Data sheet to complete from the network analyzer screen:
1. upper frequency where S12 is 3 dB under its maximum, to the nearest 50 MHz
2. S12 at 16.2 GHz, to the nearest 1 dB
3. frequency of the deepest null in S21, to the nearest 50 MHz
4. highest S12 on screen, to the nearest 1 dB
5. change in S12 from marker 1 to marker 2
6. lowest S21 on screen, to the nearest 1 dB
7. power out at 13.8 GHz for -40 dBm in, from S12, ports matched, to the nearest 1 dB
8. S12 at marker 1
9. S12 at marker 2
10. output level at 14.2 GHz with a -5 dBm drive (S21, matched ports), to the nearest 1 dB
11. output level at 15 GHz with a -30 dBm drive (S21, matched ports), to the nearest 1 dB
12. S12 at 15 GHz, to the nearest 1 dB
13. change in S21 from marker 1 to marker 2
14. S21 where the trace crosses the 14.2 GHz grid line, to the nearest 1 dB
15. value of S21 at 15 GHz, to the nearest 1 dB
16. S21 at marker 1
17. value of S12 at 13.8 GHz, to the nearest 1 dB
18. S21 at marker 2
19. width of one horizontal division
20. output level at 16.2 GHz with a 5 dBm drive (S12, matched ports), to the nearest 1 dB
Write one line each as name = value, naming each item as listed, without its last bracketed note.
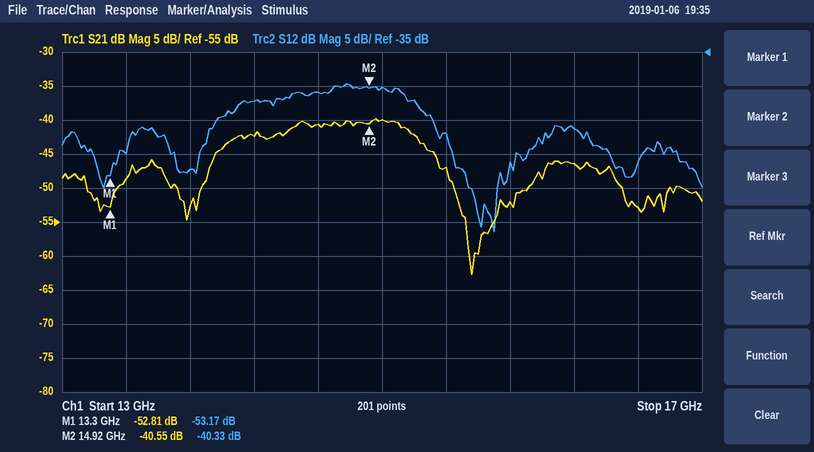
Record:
upper frequency where S12 is 3 dB under its maximum, to the nearest 50 MHz = 15.20 GHz
S12 at 16.2 GHz, to the nearest 1 dB = -46 dB
frequency of the deepest null in S21, to the nearest 50 MHz = 15.55 GHz
highest S12 on screen, to the nearest 1 dB = -40 dB
change in S12 from marker 1 to marker 2 = 12.84 dB
lowest S21 on screen, to the nearest 1 dB = -63 dB
power out at 13.8 GHz for -40 dBm in, from S12, ports matched, to the nearest 1 dB = -92 dBm
S12 at marker 1 = -53.17 dB
S12 at marker 2 = -40.33 dB
output level at 14.2 GHz with a -5 dBm drive (S21, matched ports), to the nearest 1 dB = -47 dBm
output level at 15 GHz with a -30 dBm drive (S21, matched ports), to the nearest 1 dB = -70 dBm
S12 at 15 GHz, to the nearest 1 dB = -40 dB
change in S21 from marker 1 to marker 2 = 12.26 dB
S21 where the trace crosses the 14.2 GHz grid line, to the nearest 1 dB = -42 dB
value of S21 at 15 GHz, to the nearest 1 dB = -40 dB
S21 at marker 1 = -52.81 dB
value of S12 at 13.8 GHz, to the nearest 1 dB = -52 dB
S21 at marker 2 = -40.55 dB
width of one horizontal division = 400 MHz
output level at 16.2 GHz with a 5 dBm drive (S12, matched ports), to the nearest 1 dB = -41 dBm
